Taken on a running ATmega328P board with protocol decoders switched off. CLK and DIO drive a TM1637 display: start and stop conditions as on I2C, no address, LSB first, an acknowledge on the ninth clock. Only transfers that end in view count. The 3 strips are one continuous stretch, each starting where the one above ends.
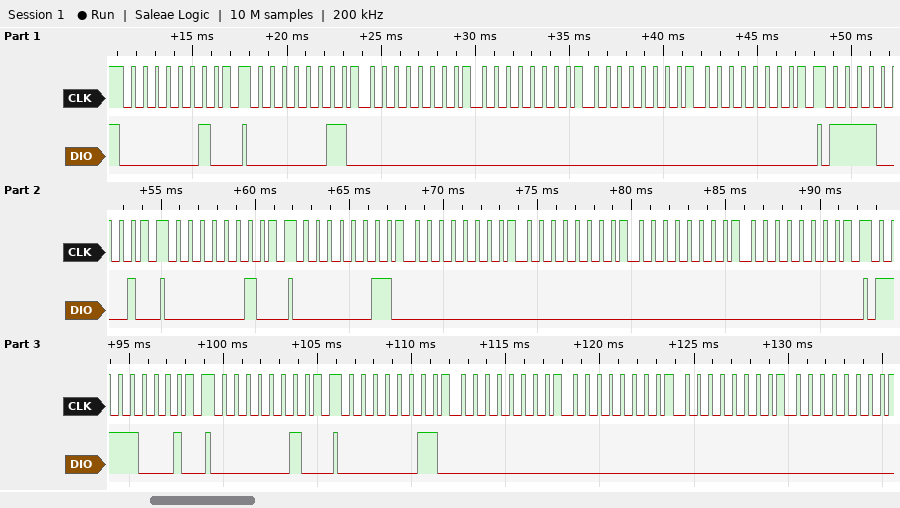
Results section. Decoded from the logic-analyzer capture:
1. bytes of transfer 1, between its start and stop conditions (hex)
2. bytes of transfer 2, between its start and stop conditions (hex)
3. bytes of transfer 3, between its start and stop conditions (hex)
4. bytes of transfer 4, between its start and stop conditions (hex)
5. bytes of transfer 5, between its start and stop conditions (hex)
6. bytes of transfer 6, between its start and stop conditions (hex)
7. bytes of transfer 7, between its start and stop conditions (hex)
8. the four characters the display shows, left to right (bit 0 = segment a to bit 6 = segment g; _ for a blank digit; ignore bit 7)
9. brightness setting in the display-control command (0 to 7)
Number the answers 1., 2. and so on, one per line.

1. 40
2. C0 00 00 00 00
3. 8F
4. 40
5. C0 00 00 00 00
6. 8F
7. 40
8. ____
9. 7
